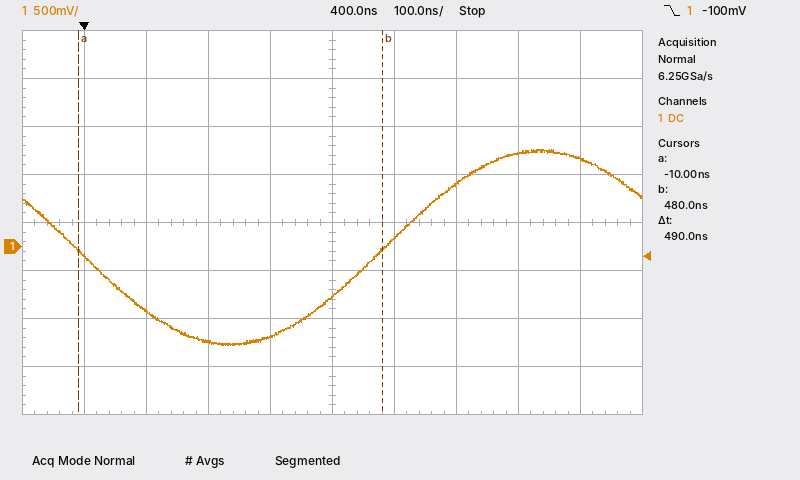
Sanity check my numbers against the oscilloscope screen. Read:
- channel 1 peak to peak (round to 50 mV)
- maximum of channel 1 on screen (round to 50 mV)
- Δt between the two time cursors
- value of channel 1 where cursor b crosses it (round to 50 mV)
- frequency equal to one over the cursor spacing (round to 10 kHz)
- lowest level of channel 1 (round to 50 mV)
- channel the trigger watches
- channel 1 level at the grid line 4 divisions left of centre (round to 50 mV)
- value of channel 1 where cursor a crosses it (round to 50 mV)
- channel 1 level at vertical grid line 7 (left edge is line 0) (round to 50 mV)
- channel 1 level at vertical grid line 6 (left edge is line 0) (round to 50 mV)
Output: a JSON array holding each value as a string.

["2.05 V", "1.00 V", "490 ns", "-50 mV", "2.04 MHz", "-1.05 V", "channel 1", "-100 mV", "-50 mV", "650 mV", "100 mV"]
